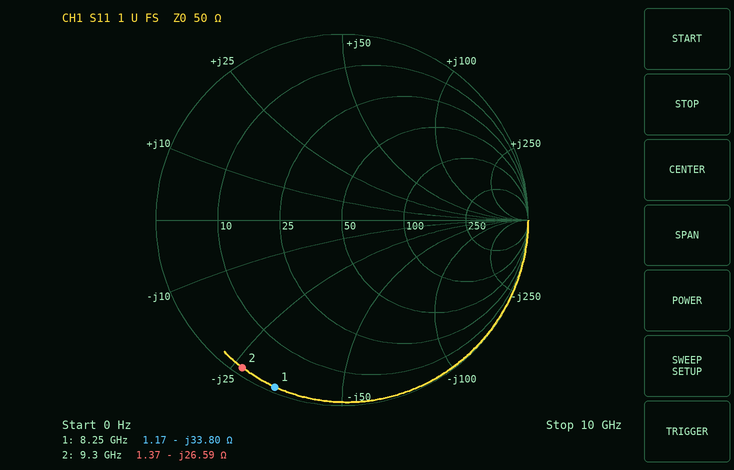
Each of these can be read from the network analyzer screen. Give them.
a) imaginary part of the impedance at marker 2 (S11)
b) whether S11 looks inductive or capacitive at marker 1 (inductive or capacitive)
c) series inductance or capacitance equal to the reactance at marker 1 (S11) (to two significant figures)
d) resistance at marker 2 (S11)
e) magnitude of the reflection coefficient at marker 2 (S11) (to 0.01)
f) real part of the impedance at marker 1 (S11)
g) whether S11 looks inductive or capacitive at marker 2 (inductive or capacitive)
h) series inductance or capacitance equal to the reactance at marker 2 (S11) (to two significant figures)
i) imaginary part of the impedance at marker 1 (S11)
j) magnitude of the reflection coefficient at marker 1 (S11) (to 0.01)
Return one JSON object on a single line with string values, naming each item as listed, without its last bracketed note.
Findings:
{"imaginary part of the impedance at marker 2": "-26.59 Ω", "whether S11 looks inductive or capacitive at marker 1": "capacitive", "series inductance or capacitance equal to the reactance at marker 1 (S11)": "570 fF", "resistance at marker 2": "1.37 Ω", "magnitude of the reflection coefficient at marker 2 (S11)": "0.96", "real part of the impedance at marker 1": "1.17 Ω", "whether S11 looks inductive or capacitive at marker 2": "capacitive", "series inductance or capacitance equal to the reactance at marker 2 (S11)": "640 fF", "imaginary part of the impedance at marker 1": "-33.80 Ω", "magnitude of the reflection coefficient at marker 1 (S11)": "0.97"}
